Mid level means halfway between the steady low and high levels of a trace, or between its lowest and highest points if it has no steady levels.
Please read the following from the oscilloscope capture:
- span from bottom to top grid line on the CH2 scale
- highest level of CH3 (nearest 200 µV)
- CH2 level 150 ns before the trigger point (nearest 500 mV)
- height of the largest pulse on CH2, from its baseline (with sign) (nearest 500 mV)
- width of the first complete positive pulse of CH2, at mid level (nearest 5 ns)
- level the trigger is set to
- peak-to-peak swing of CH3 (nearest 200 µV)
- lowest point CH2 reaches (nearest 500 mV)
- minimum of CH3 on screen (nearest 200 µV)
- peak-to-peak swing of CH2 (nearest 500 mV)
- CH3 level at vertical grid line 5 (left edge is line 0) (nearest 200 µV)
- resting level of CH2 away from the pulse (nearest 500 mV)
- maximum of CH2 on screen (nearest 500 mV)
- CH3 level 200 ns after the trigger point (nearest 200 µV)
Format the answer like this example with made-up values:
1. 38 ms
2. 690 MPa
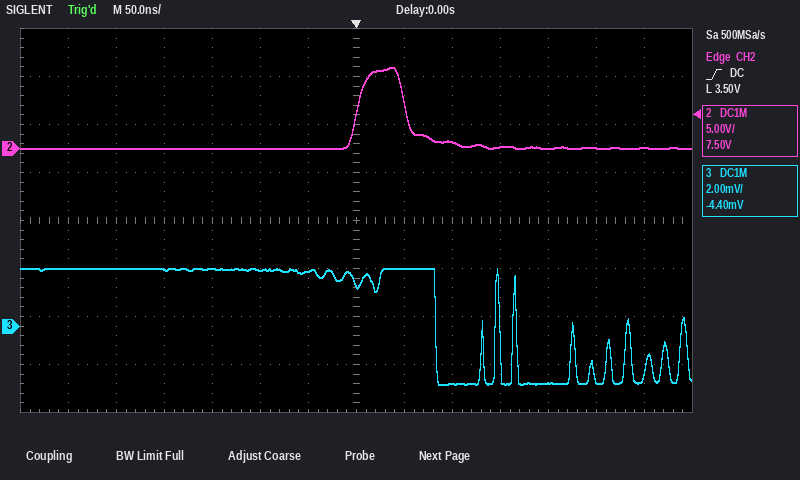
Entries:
1. 40 V
2. 2.4 mV
3. 0.0 V
4. +8.5 V
5. 50 ns
6. 3.50 V
7. 4.8 mV
8. 0.0 V
9. -2.4 mV
10. 8.5 V
11. 2.4 mV
12. 0.0 V
13. 8.5 V
14. -2.4 mV
